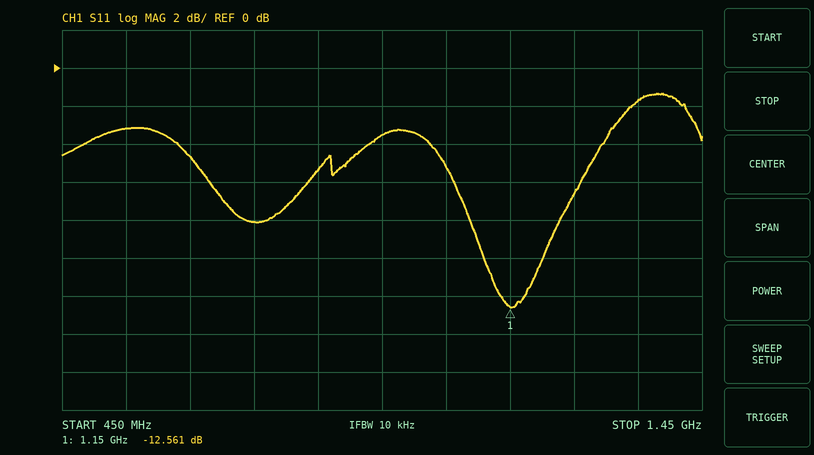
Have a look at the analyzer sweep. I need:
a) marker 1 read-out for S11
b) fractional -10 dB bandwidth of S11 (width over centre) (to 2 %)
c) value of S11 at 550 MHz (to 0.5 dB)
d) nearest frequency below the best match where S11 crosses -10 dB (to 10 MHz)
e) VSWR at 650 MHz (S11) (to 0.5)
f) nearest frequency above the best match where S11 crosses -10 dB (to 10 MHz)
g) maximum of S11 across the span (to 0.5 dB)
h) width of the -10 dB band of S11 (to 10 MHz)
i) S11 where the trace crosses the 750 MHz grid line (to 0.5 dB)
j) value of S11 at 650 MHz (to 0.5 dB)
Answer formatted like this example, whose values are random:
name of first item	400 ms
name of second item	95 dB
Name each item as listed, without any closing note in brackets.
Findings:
marker 1 read-out for S11	-12.561 dB
fractional -10 dB bandwidth of S11 (width over centre)	8 %
value of S11 at 550 MHz	-3.0 dB
nearest frequency below the best match where S11 crosses -10 dB	1.11 GHz
VSWR at 650 MHz (S11)	4.0
nearest frequency above the best match where S11 crosses -10 dB	1.20 GHz
maximum of S11 across the span	-1.5 dB
width of the -10 dB band of S11	90 MHz
S11 where the trace crosses the 750 MHz grid line	-8.0 dB
value of S11 at 650 MHz	-4.5 dB
